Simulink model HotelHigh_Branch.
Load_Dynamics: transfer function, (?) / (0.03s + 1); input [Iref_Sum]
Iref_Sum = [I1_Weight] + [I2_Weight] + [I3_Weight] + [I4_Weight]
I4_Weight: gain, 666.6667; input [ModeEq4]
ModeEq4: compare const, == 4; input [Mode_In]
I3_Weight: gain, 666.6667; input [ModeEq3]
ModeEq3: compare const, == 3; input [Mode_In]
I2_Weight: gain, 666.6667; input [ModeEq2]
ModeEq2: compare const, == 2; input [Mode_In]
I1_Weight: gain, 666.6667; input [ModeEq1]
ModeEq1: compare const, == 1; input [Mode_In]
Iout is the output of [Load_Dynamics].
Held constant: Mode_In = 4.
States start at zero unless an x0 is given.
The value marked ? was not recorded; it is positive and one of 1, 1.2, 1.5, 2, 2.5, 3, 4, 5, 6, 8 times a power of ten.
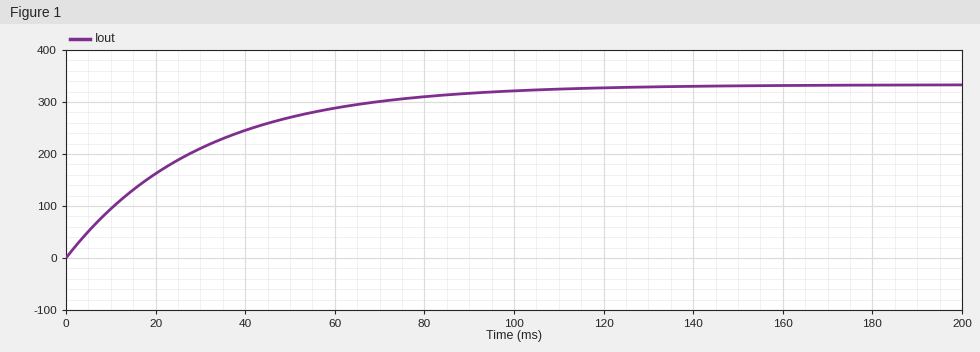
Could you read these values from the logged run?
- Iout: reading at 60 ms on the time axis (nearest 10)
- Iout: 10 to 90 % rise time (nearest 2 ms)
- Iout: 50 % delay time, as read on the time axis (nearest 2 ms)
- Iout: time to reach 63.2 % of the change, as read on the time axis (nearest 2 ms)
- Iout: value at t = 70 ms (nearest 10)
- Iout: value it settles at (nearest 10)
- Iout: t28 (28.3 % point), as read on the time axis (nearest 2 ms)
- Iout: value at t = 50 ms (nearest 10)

290
66 ms
20 ms
30 ms
300
330
10 ms
270
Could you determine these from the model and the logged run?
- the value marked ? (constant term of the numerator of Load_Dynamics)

0.5
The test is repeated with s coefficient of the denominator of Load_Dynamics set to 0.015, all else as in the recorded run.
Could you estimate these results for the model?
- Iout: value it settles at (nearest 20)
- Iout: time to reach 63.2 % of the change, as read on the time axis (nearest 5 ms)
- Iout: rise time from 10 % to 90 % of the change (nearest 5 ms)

340
15 ms
35 ms
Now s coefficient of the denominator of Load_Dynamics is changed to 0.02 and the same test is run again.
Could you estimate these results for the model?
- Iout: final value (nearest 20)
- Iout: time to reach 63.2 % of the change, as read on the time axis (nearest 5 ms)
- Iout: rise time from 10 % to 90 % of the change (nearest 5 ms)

340
20 ms
45 ms
